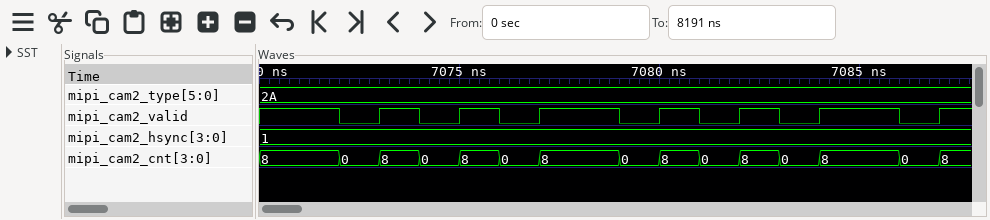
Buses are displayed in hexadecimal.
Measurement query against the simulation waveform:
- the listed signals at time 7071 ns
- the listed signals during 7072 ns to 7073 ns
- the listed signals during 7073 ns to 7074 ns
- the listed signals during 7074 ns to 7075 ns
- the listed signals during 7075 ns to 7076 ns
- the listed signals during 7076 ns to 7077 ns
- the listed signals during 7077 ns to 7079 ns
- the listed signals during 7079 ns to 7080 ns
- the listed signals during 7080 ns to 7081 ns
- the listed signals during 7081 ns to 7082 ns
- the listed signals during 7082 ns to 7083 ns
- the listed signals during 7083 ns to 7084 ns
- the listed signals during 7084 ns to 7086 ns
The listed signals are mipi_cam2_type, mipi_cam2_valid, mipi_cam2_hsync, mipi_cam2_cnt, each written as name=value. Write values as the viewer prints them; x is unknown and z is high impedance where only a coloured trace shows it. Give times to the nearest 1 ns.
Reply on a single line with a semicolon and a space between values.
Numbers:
mipi_cam2_type=2A, mipi_cam2_valid=1, mipi_cam2_hsync=1, mipi_cam2_cnt=8; mipi_cam2_type=2A, mipi_cam2_valid=0, mipi_cam2_hsync=1, mipi_cam2_cnt=0; mipi_cam2_type=2A, mipi_cam2_valid=1, mipi_cam2_hsync=1, mipi_cam2_cnt=8; mipi_cam2_type=2A, mipi_cam2_valid=0, mipi_cam2_hsync=1, mipi_cam2_cnt=0; mipi_cam2_type=2A, mipi_cam2_valid=1, mipi_cam2_hsync=1, mipi_cam2_cnt=8; mipi_cam2_type=2A, mipi_cam2_valid=0, mipi_cam2_hsync=1, mipi_cam2_cnt=0; mipi_cam2_type=2A, mipi_cam2_valid=1, mipi_cam2_hsync=1, mipi_cam2_cnt=8; mipi_cam2_type=2A, mipi_cam2_valid=0, mipi_cam2_hsync=1, mipi_cam2_cnt=0; mipi_cam2_type=2A, mipi_cam2_valid=1, mipi_cam2_hsync=1, mipi_cam2_cnt=8; mipi_cam2_type=2A, mipi_cam2_valid=0, mipi_cam2_hsync=1, mipi_cam2_cnt=0; mipi_cam2_type=2A, mipi_cam2_valid=1, mipi_cam2_hsync=1, mipi_cam2_cnt=8; mipi_cam2_type=2A, mipi_cam2_valid=0, mipi_cam2_hsync=1, mipi_cam2_cnt=0; mipi_cam2_type=2A, mipi_cam2_valid=1, mipi_cam2_hsync=1, mipi_cam2_cnt=8
